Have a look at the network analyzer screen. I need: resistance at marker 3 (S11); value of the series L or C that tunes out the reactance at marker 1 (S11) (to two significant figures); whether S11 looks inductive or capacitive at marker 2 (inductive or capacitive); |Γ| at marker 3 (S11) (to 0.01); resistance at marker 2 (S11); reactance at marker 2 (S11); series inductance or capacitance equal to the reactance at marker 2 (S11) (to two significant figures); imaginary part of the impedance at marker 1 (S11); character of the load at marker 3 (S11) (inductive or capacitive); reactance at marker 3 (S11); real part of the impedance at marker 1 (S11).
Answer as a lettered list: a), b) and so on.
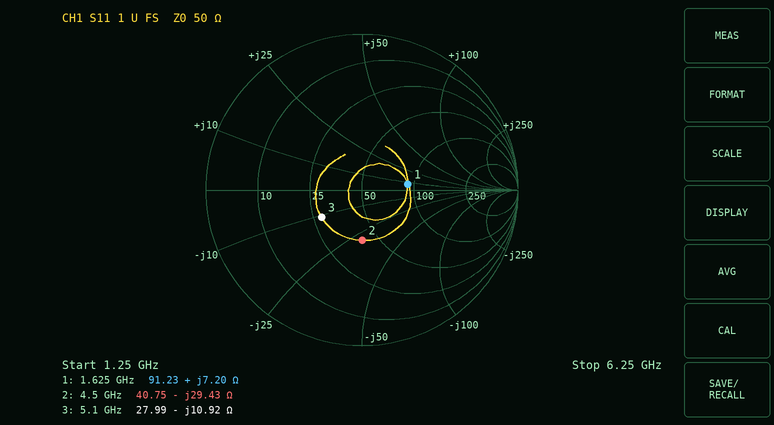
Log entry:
a) 27.99 Ω
b) 14 pF
c) capacitive
d) 0.31
e) 40.75 Ω
f) -29.43 Ω
g) 1.2 pF
h) +7.20 Ω
i) capacitive
j) -10.92 Ω
k) 91.23 Ω
